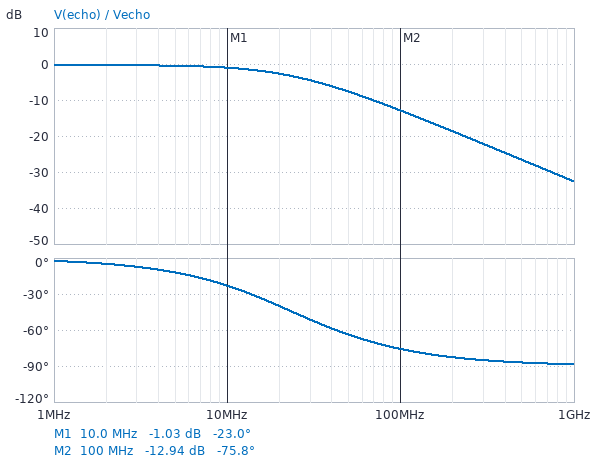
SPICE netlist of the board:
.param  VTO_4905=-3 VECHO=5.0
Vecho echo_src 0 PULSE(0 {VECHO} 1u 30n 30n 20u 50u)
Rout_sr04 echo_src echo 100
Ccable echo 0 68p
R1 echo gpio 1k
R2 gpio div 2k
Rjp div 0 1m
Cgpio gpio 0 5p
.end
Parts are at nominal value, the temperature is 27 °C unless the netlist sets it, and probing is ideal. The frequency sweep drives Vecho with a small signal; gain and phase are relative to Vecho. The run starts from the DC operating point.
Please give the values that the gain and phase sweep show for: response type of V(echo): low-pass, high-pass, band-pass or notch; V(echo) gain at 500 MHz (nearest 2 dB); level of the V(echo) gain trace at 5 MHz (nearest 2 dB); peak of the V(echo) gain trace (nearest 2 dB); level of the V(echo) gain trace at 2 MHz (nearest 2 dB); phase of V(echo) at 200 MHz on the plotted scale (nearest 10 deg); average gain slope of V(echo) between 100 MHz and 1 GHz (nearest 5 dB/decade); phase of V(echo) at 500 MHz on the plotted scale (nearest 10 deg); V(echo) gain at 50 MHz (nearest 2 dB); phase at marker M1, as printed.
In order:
low-pass
-26 dB
0 dB
0 dB
0 dB
-80 deg
-20 dB/decade
-90 deg
-8 dB
-23.0 deg
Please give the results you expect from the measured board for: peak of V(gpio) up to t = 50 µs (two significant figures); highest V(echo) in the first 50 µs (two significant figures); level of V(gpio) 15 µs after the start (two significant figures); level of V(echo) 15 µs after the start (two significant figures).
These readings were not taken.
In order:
3.2 V
4.8 V
3.2 V
4.8 V
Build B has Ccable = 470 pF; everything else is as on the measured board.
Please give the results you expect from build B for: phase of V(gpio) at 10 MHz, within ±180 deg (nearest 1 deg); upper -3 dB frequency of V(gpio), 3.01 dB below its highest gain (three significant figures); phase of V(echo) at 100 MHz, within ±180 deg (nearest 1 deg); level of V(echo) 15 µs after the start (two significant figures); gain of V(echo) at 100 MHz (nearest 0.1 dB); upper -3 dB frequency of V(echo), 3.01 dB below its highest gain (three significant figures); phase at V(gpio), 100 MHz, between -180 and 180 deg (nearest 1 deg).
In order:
-83 deg
3.46 MHz
-88 deg
4.8 V
-29.4 dB
3.48 MHz
-152 deg
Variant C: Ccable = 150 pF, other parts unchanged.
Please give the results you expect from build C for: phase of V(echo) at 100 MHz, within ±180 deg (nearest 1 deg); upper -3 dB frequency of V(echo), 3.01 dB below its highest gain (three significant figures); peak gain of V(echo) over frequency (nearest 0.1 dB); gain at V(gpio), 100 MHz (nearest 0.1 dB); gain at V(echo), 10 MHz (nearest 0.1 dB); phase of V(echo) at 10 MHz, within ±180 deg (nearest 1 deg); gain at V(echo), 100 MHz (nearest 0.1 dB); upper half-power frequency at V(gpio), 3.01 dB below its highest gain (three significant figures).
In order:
-83 deg
10.8 MHz
-0.3 dB
-30.4 dB
-3.0 dB
-43 deg
-19.6 dB
10.3 MHz
